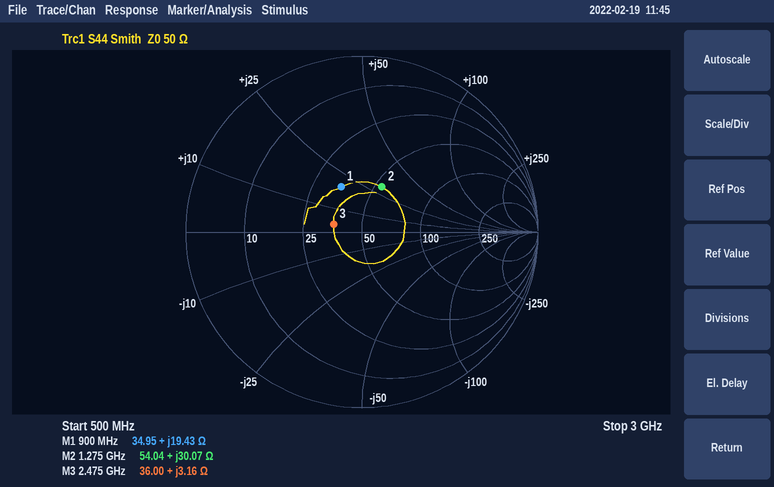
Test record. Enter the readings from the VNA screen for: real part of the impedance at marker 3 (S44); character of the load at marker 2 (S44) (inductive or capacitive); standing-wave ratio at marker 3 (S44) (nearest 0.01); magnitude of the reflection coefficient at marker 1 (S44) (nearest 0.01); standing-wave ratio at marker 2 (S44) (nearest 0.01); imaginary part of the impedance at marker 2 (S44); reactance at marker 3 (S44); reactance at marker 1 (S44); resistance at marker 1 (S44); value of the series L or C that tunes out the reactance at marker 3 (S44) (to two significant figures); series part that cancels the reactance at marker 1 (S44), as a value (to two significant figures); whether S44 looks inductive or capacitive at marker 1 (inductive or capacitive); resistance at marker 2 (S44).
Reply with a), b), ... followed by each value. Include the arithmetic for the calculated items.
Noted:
a) 36.00 Ω
b) inductive
c) 1.40
d) 0.28
e) 1.78
f) +30.07 Ω
g) +3.16 Ω
h) +19.43 Ω
i) 34.95 Ω
j) C = 1/(2π × 2.475 GHz × 3.16 Ω) ≈ 20 pF
k) C = 1/(2π × 900 MHz × 19.43 Ω) ≈ 9.1 pF
l) inductive
m) 54.04 Ω
